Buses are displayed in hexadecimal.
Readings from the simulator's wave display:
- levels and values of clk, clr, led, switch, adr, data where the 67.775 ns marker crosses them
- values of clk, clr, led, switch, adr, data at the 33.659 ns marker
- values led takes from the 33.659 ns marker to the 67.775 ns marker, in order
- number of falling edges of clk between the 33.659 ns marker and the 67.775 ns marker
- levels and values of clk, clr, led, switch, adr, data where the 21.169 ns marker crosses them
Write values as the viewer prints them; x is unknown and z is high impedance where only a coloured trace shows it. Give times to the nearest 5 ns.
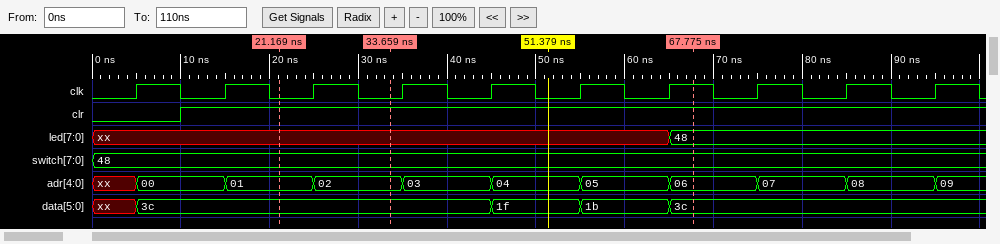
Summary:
clk=1, clr=1, led=48, switch=48, adr=06, data=3c
clk=0, clr=1, led=xx, switch=48, adr=02, data=3c
xx, 48
3
clk=0, clr=1, led=xx, switch=48, adr=01, data=3c
